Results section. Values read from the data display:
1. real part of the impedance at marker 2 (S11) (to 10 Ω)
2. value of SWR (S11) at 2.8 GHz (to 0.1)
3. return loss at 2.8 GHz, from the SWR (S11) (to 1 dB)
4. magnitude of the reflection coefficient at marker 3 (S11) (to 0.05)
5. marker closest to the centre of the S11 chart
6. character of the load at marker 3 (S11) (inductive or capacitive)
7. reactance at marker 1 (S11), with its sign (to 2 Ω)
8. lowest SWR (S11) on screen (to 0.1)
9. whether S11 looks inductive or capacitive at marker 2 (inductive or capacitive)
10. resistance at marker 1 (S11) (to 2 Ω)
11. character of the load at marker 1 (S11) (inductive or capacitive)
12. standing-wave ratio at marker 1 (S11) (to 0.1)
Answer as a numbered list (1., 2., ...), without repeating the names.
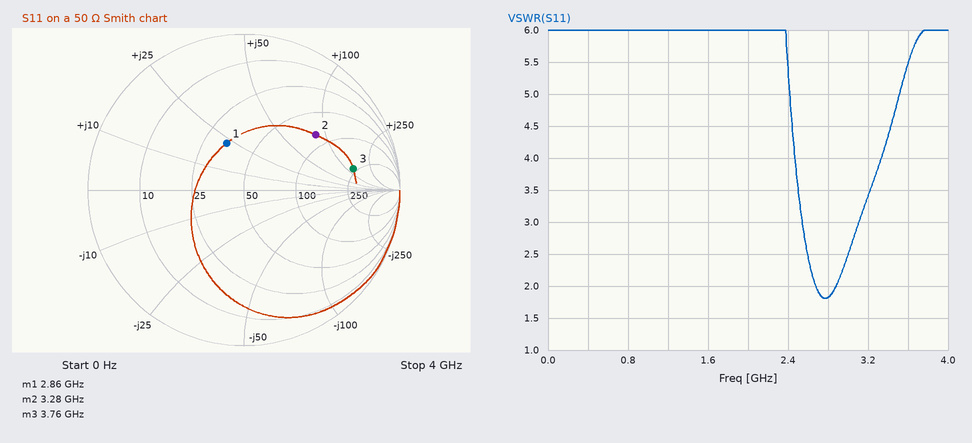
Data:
1. 80 Ω
2. 1.8
3. 11 dB
4. 0.70
5. marker 1
6. inductive
7. +22 Ω
8. 1.8
9. inductive
10. 34 Ω
11. inductive
12. 1.9
